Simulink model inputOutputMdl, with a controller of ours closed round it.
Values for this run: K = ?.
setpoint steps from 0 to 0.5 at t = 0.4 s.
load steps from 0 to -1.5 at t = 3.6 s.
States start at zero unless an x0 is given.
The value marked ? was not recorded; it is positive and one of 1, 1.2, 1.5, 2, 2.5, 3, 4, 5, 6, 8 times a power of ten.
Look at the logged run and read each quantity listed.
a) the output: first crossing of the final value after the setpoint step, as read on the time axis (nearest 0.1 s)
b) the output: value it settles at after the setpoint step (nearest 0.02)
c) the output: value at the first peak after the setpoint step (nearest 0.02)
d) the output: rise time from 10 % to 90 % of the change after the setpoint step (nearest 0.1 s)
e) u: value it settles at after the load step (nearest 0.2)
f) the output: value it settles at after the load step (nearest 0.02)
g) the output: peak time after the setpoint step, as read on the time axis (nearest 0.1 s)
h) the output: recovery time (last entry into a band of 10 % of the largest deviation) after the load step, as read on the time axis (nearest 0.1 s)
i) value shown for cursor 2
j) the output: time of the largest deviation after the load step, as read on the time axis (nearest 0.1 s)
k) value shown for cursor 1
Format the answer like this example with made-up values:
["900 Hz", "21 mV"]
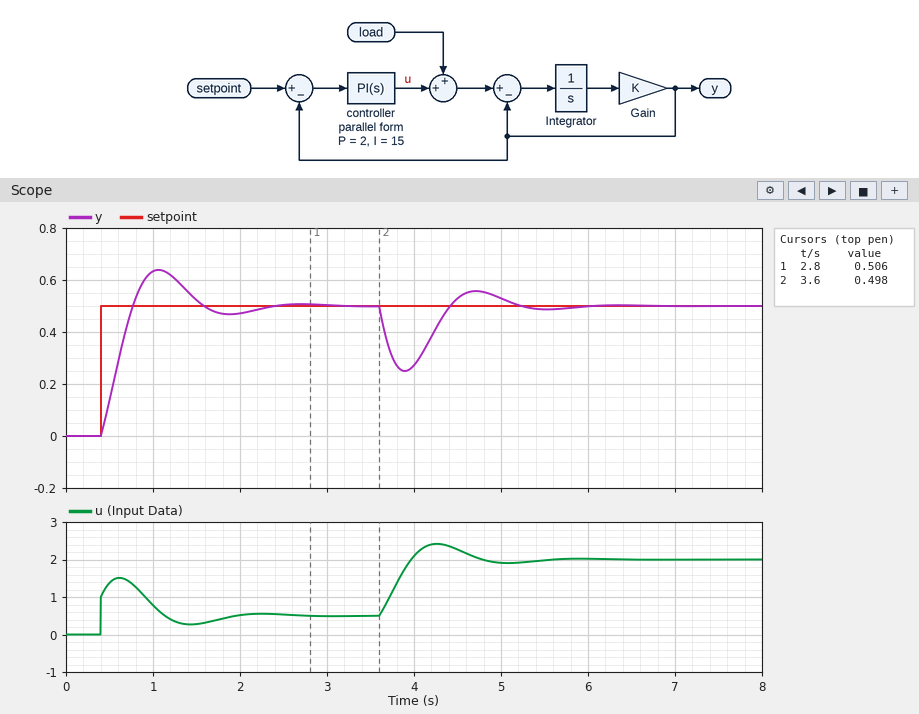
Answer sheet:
["0.8 s", "0.50", "0.64", "0.3 s", "2.0", "0.50", "1.1 s", "5.0 s", "0.498", "3.9 s", "0.506"]
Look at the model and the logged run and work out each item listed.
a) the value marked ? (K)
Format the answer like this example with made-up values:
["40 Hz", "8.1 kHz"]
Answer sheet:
["1.2"]
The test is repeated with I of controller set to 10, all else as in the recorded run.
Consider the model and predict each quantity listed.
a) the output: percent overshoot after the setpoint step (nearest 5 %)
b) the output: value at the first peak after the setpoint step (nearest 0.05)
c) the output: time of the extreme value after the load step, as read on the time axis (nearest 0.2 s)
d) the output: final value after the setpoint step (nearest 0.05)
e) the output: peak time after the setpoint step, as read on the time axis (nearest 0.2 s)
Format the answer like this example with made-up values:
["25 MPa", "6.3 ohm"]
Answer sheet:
["20 %", "0.60", "4.0 s", "0.50", "1.2 s"]
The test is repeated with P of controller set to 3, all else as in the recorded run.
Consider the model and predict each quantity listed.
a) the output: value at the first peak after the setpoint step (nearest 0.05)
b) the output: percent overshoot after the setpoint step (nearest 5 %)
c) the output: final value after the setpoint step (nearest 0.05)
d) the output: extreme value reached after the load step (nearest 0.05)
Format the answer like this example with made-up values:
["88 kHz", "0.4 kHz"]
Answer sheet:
["0.60", "20 %", "0.50", "0.30"]
